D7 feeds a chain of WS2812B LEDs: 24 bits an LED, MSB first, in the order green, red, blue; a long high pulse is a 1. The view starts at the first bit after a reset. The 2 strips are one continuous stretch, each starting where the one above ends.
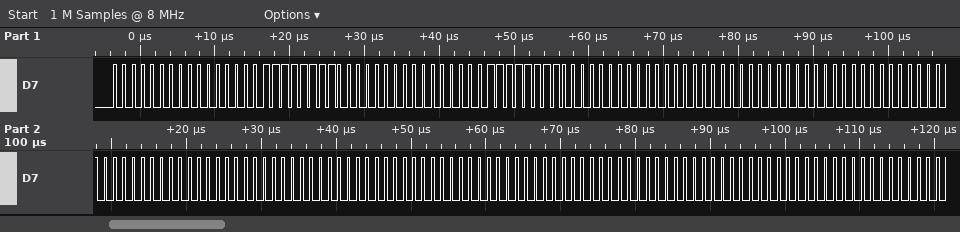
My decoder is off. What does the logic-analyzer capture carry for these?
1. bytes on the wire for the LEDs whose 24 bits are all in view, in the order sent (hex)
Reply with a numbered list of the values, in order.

1. 00 00 FF 00 00 FF 00 00 00 00 00 00 00 00 00 00 00 00 00 00 00
